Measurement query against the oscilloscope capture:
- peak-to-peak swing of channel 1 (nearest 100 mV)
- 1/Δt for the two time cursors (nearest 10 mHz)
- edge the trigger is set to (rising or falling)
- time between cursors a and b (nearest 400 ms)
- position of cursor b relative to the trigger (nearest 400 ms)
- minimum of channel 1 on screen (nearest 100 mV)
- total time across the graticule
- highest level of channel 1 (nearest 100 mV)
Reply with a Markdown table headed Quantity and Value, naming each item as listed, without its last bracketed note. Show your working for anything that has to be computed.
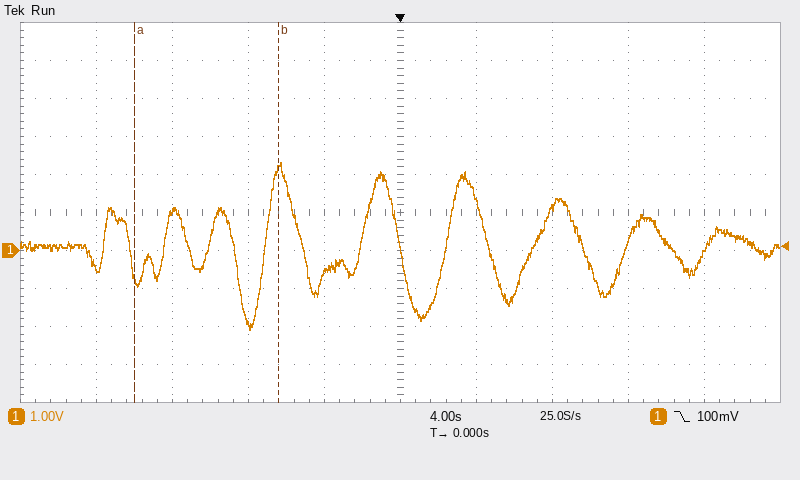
| Quantity | Value |
|---|---|
| peak-to-peak swing of channel 1 | 2.3 V − (-2.1 V) = 4.4 V |
| 1/Δt for the two time cursors | 1 / 7.6 s ≈ 130 mHz |
| edge the trigger is set to | falling |
| time between cursors a and b | 7.6 s |
| position of cursor b relative to the trigger | -6.4 s |
| minimum of channel 1 on screen | -2.1 V |
| total time across the graticule | 40 s |
| highest level of channel 1 | 2.3 V |
